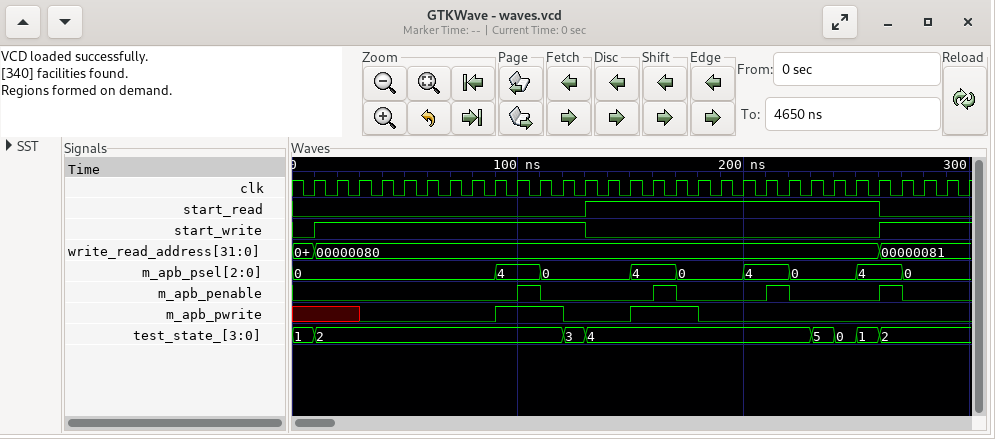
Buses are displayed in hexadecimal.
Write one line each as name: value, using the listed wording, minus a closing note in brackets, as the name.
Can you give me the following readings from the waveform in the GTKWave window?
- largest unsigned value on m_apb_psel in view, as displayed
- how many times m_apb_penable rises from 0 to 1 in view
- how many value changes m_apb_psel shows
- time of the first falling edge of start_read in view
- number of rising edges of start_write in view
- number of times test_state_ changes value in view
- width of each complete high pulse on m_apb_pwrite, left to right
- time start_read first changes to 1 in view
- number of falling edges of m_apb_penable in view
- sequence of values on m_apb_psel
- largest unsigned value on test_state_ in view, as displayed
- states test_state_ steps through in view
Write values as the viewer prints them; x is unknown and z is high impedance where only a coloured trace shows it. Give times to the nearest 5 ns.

largest unsigned value on m_apb_psel in view, as displayed: 4
how many times m_apb_penable rises from 0 to 1 in view: 4
how many value changes m_apb_psel shows: 8
time of the first falling edge of start_read in view: 260 ns
number of rising edges of start_write in view: 2
number of times test_state_ changes value in view: 7
width of each complete high pulse on m_apb_pwrite, left to right: 30 ns, 30 ns
time start_read first changes to 1 in view: 130 ns
number of falling edges of m_apb_penable in view: 4
sequence of values on m_apb_psel: 0, 4, 0, 4, 0, 4, 0, 4, 0
largest unsigned value on test_state_ in view, as displayed: 5
states test_state_ steps through in view: 1, 2, 3, 4, 5, 0, 1, 2
